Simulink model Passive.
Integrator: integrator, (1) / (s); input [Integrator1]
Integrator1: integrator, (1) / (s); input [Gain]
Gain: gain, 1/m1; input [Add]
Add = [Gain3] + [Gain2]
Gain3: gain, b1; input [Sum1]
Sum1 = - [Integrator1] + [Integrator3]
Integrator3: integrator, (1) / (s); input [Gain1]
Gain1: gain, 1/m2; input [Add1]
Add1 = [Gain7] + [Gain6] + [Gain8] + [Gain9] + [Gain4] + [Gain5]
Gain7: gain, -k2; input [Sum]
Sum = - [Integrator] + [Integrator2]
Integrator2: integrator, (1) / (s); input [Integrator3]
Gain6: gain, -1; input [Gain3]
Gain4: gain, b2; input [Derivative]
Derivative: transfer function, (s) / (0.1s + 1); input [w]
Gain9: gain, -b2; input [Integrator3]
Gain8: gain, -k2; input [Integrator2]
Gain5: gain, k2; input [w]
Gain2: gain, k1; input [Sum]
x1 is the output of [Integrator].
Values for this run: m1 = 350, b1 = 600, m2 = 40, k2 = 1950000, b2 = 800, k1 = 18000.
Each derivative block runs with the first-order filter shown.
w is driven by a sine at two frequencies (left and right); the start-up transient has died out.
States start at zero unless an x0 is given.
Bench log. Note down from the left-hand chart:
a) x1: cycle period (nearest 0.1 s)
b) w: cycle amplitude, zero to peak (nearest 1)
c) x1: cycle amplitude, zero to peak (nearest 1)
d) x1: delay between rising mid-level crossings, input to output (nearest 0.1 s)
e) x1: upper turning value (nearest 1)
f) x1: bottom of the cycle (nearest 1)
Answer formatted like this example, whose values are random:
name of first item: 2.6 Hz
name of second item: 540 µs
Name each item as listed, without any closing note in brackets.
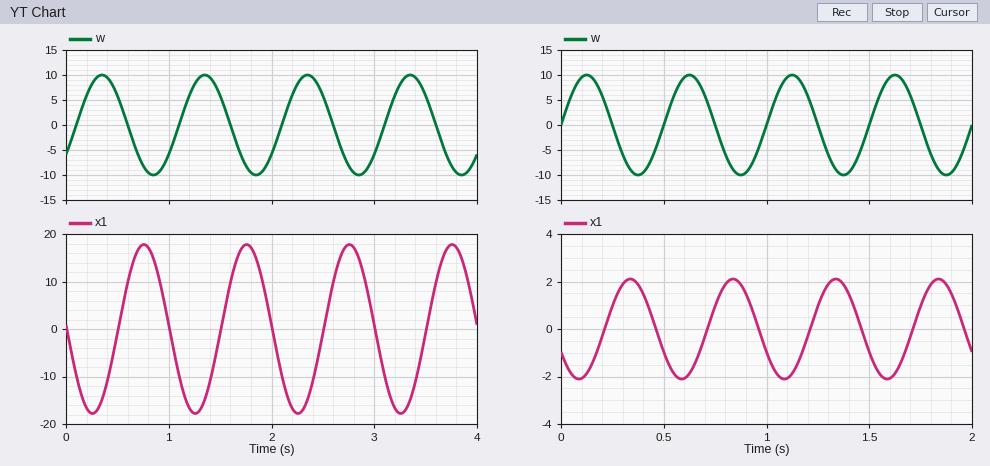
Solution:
x1: cycle period: 1.0 s
w: cycle amplitude, zero to peak: 10
x1: cycle amplitude, zero to peak: 18
x1: delay between rising mid-level crossings, input to output: 0.4 s
x1: upper turning value: 18
x1: bottom of the cycle: -18
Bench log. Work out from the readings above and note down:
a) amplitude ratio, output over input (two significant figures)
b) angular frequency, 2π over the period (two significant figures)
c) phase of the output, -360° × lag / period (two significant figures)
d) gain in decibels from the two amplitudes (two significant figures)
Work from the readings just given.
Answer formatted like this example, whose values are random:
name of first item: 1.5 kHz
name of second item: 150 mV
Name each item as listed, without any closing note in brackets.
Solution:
amplitude ratio, output over input: 1.8
angular frequency, 2π over the period: 6.3 rad/s
phase of the output, -360° × lag / period: -140°
gain in decibels from the two amplitudes: 5.1 dB
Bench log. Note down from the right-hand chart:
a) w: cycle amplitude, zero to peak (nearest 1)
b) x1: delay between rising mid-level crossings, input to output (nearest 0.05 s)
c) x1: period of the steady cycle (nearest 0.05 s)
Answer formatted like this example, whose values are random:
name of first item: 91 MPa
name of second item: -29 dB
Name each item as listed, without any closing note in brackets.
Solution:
w: cycle amplitude, zero to peak: 10
x1: delay between rising mid-level crossings, input to output: 0.20 s
x1: period of the steady cycle: 0.50 s
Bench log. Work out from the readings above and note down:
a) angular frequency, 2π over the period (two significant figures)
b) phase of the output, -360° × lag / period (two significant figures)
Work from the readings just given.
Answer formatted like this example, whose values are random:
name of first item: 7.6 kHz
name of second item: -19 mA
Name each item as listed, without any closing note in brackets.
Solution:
angular frequency, 2π over the period: 13 rad/s
phase of the output, -360° × lag / period: -140°
